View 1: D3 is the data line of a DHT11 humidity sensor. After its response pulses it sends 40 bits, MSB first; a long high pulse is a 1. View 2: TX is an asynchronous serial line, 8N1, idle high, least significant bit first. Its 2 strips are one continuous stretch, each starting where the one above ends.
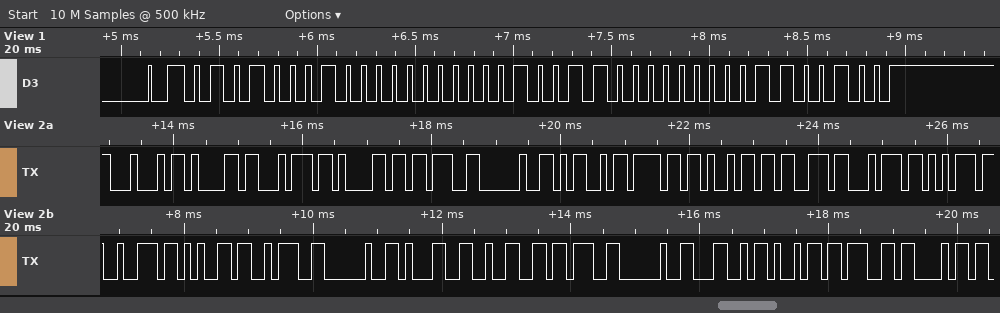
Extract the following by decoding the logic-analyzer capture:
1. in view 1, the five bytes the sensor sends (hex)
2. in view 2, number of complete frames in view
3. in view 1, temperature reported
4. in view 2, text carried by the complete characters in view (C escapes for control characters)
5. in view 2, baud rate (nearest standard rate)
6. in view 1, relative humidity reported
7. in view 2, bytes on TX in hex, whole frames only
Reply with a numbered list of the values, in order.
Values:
1. 51 00 13 00 64
2. 24
3. 19.0 °C
4. "Data; Moisture: 12; Ligh"
5. 9600 baud
6. 81 %
7. 44 61 74 61 3B 20 4D 6F 69 73 74 75 72 65 3A 20 31 32 3B 20 4C 69 67 68
